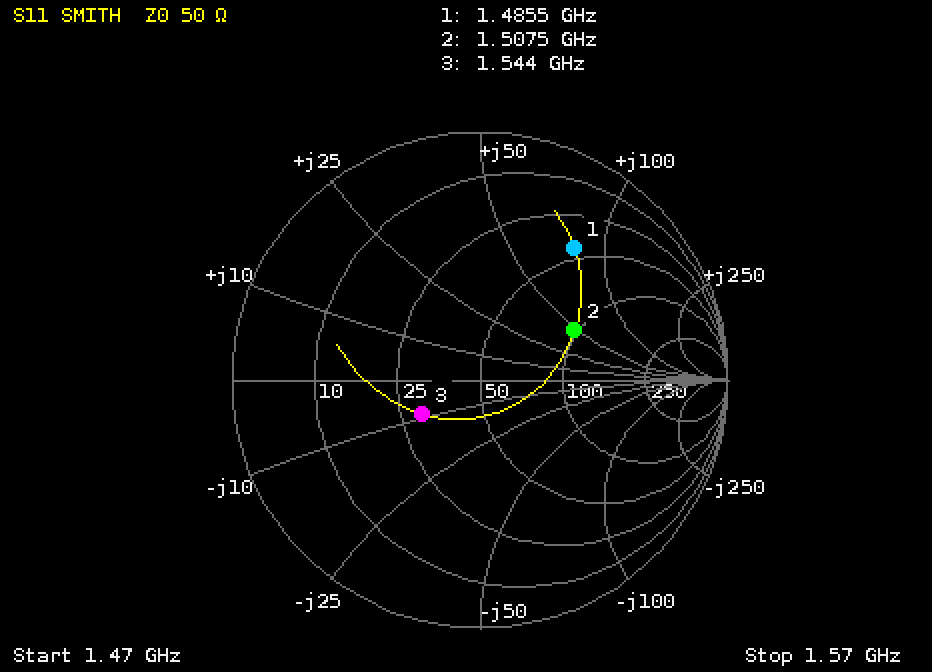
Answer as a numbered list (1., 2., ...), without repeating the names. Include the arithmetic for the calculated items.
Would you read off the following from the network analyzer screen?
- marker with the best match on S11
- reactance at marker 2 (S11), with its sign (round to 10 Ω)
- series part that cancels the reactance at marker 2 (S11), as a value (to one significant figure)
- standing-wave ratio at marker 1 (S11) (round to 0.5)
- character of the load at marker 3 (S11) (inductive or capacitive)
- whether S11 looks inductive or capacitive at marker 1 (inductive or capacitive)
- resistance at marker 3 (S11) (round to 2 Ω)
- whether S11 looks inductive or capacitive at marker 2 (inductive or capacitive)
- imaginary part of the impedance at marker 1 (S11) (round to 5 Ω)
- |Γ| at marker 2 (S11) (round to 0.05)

1. marker 3
2. +50 Ω
3. C = 1/(2π × 1.5075 GHz × 50 Ω) ≈ 2 pF
4. 5.0
5. capacitive
6. inductive
7. 30 Ω
8. inductive
9. +80 Ω
10. 0.45
